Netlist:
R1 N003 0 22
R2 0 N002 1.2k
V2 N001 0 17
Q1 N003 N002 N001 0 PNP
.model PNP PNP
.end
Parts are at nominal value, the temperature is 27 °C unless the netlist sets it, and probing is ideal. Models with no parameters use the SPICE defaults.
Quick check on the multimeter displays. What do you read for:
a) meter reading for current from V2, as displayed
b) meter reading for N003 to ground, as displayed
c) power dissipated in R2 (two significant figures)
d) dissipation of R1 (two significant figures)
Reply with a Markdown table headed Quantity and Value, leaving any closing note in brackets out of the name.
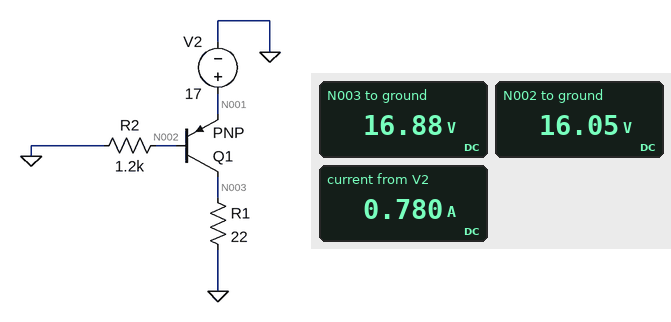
| Quantity | Value |
|---|---|
| meter reading for current from V2, as displayed | 0.780 A |
| meter reading for N003 to ground, as displayed | 16.88 V |
| power dissipated in R2 | 210 mW |
| dissipation of R1 | 13 W |
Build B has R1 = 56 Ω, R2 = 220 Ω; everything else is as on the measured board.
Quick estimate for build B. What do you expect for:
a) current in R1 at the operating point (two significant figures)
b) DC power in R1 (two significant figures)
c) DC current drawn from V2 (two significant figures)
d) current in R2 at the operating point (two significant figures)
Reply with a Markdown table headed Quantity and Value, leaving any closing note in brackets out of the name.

| Quantity | Value |
|---|---|
| current in R1 at the operating point | 300 mA |
| DC power in R1 | 5.1 W |
| DC current drawn from V2 | 380 mA |
| current in R2 at the operating point | 73 mA |
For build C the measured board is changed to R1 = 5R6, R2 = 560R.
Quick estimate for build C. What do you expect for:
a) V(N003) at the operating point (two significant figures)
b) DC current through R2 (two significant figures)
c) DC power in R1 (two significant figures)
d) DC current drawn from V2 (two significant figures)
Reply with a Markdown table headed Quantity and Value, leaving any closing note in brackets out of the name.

| Quantity | Value |
|---|---|
| V(N003) at the operating point | 16 V |
| DC current through R2 | 29 mA |
| DC power in R1 | 46 W |
| DC current drawn from V2 | 2.9 A |
